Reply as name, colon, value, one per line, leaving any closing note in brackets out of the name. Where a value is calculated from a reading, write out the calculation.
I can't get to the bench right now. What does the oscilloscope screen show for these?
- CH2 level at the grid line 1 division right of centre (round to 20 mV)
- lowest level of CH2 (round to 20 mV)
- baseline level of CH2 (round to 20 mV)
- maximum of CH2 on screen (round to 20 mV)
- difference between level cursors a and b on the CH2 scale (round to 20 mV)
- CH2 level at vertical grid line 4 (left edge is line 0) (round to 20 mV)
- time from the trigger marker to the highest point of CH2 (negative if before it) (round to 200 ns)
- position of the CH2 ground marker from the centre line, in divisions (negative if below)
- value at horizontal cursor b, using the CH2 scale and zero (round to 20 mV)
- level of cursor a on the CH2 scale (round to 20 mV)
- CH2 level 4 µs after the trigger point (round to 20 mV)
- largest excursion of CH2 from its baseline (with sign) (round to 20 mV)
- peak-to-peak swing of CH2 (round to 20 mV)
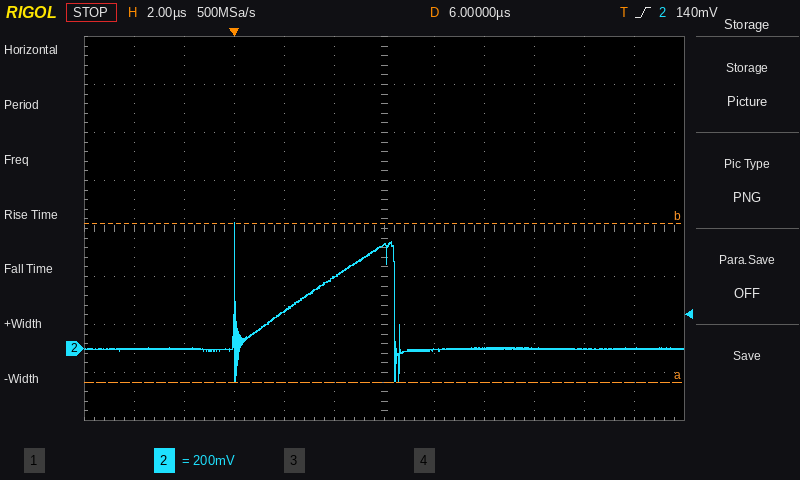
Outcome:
CH2 level at the grid line 1 division right of centre: 0 mV
lowest level of CH2: -140 mV
baseline level of CH2: 0 mV
maximum of CH2 on screen: 520 mV
difference between level cursors a and b on the CH2 scale: 660 mV
CH2 level at vertical grid line 4 (left edge is line 0): 160 mV
time from the trigger marker to the highest point of CH2 (negative if before it): 0.0 µs
position of the CH2 ground marker from the centre line, in divisions: -2.5 div
value at horizontal cursor b, using the CH2 scale and zero: 520 mV
level of cursor a on the CH2 scale: -140 mV
CH2 level 4 µs after the trigger point: 300 mV
largest excursion of CH2 from its baseline (with sign): 520 mV − (0 mV) = +520 mV
peak-to-peak swing of CH2: 520 mV − (-140 mV) = 660 mV
